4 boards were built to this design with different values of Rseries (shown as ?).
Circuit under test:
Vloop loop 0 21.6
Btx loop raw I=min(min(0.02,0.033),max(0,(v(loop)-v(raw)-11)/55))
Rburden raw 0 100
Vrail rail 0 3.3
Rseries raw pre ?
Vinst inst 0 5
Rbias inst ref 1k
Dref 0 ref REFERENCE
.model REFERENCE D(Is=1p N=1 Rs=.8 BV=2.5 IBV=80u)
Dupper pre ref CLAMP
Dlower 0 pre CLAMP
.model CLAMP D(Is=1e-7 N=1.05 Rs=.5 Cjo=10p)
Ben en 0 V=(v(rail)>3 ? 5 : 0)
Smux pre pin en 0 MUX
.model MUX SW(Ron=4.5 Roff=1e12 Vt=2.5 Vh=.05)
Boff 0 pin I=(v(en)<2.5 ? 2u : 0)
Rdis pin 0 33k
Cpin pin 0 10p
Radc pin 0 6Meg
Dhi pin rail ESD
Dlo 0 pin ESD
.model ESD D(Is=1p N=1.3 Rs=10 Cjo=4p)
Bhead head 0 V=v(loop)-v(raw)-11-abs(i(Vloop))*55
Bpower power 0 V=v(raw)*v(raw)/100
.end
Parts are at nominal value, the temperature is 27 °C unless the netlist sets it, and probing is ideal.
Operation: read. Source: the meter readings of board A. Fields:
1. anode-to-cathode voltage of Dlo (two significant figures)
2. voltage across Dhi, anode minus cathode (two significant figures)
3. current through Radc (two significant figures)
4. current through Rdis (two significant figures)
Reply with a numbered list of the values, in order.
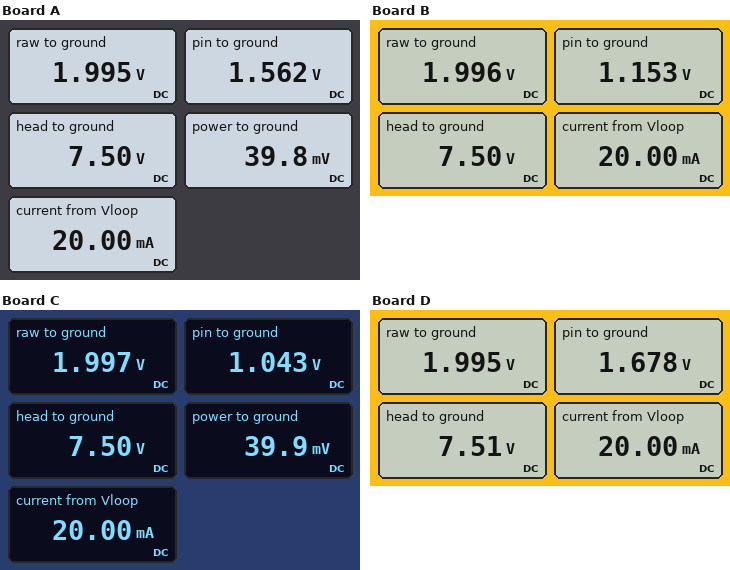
1. -1.6 V
2. -1.7 V
3. 260 nA
4. 47 µA
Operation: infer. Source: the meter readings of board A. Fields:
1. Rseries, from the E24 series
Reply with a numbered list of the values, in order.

1. 9.1 kΩ
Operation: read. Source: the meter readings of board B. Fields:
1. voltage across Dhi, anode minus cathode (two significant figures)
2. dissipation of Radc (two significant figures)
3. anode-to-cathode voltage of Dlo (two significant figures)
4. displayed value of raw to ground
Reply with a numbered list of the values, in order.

1. -2.1 V
2. 220 nW
3. -1.2 V
4. 1.996 V
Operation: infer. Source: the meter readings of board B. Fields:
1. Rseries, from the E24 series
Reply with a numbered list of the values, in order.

1. 24 kΩ
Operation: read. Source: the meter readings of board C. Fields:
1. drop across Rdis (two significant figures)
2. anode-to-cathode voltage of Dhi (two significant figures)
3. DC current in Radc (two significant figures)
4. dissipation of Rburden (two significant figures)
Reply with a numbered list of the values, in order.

1. 1.0 V
2. -2.3 V
3. 170 nA
4. 40 mW
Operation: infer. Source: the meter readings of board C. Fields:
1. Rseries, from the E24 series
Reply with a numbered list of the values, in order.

1. 30 kΩ
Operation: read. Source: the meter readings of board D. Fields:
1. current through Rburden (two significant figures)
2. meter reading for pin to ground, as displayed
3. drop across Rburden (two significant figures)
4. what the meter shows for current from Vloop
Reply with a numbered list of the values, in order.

1. 20 mA
2. 1.678 V
3. 2.0 V
4. 20.00 mA
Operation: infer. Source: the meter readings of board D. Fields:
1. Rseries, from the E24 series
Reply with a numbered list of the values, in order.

1. 6.2 kΩ
